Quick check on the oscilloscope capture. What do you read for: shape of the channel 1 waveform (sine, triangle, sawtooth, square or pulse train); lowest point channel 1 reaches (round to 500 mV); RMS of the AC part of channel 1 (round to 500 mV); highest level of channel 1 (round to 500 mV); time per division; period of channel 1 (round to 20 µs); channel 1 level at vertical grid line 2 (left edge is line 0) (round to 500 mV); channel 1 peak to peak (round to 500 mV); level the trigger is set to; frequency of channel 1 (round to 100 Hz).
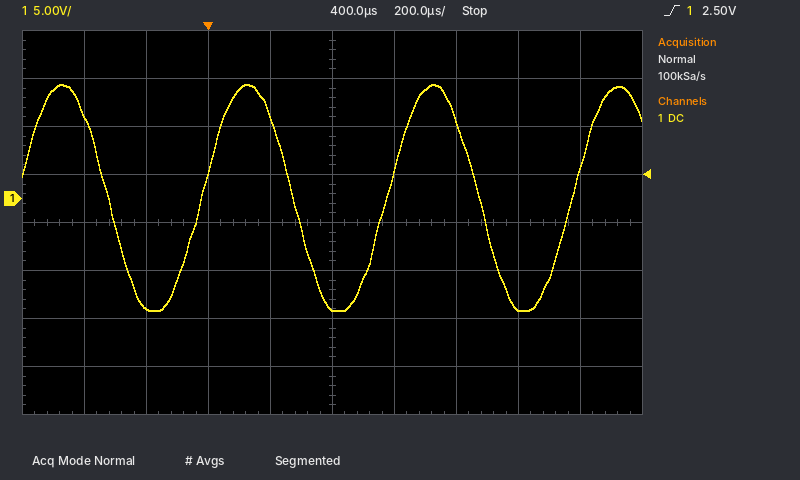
sine
-11.5 V
8.5 V
12.0 V
200 µs
600 µs
-11.5 V
23.5 V
2.50 V
1.7 kHz
